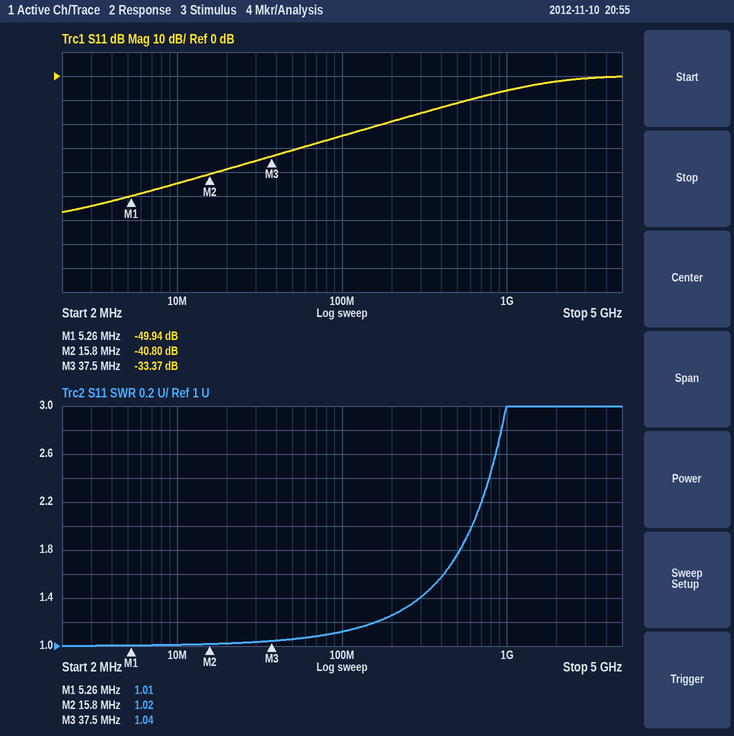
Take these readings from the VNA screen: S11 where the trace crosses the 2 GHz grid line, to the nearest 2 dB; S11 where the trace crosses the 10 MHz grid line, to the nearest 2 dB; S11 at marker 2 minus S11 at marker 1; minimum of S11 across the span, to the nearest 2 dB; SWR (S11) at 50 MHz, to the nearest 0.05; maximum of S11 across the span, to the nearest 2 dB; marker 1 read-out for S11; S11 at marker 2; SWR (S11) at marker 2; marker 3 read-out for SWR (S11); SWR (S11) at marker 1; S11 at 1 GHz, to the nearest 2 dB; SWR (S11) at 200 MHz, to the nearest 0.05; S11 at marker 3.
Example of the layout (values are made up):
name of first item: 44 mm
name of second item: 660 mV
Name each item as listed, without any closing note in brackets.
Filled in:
S11 where the trace crosses the 2 GHz grid line, to the nearest 2 dB: -2 dB
S11 where the trace crosses the 10 MHz grid line, to the nearest 2 dB: -44 dB
S11 at marker 2 minus S11 at marker 1: 9.14 dB
minimum of S11 across the span, to the nearest 2 dB: -56 dB
SWR (S11) at 50 MHz, to the nearest 0.05: 1.05
maximum of S11 across the span, to the nearest 2 dB: 0 dB
marker 1 read-out for S11: -49.94 dB
S11 at marker 2: -40.80 dB
SWR (S11) at marker 2: 1.02
marker 3 read-out for SWR: 1.04
SWR (S11) at marker 1: 1.01
S11 at 1 GHz, to the nearest 2 dB: -6 dB
SWR (S11) at 200 MHz, to the nearest 0.05: 1.25
S11 at marker 3: -33.37 dB
